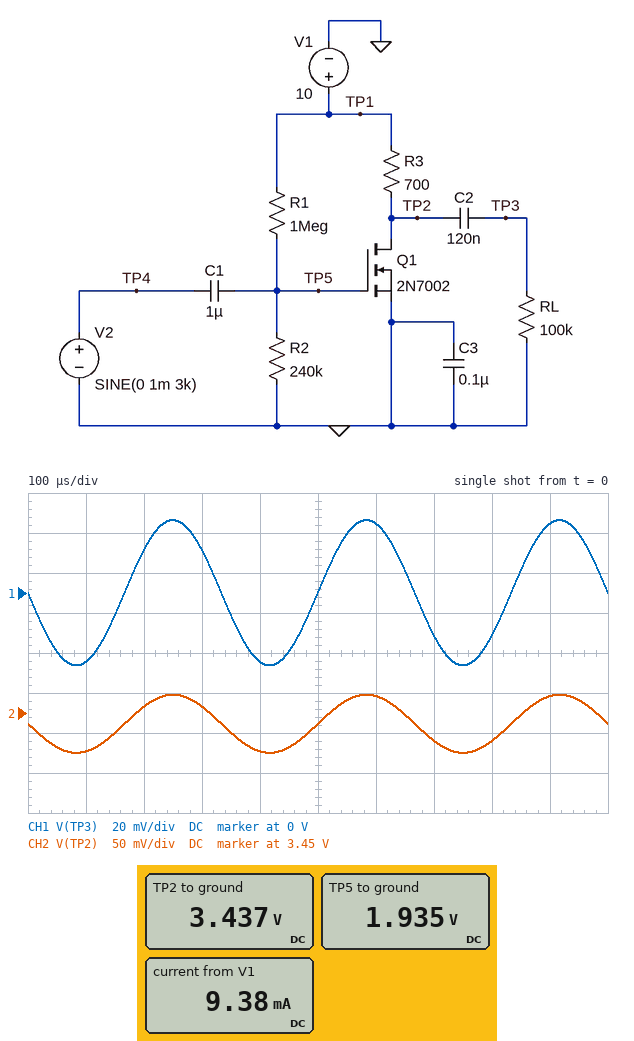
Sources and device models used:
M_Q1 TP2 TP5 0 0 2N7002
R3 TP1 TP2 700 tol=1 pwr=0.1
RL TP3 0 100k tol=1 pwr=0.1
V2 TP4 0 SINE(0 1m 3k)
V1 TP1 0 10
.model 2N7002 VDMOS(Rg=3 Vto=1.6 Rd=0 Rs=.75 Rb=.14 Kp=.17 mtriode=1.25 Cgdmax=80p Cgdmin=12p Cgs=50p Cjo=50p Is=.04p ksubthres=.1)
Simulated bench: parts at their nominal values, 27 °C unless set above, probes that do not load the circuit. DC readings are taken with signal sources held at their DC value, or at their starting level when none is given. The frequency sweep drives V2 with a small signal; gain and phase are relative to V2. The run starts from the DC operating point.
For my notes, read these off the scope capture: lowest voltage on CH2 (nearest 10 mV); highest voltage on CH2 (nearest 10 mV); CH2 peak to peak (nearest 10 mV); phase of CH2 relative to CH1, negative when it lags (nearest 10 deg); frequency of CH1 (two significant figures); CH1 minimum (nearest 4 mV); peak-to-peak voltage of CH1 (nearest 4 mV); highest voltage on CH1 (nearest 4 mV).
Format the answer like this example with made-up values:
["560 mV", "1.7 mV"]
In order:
["3.40 V", "3.47 V", "70 mV", "0 deg", "3.0 kHz", "-36 mV", "72 mV", "36 mV"]
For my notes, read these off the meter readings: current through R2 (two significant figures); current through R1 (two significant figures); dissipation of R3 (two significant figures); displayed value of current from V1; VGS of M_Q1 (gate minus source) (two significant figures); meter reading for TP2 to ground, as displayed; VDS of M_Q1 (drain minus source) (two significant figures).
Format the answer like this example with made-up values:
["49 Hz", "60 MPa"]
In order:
["8.1 µA", "8.1 µA", "62 mW", "9.38 mA", "1.9 V", "3.437 V", "3.4 V"]
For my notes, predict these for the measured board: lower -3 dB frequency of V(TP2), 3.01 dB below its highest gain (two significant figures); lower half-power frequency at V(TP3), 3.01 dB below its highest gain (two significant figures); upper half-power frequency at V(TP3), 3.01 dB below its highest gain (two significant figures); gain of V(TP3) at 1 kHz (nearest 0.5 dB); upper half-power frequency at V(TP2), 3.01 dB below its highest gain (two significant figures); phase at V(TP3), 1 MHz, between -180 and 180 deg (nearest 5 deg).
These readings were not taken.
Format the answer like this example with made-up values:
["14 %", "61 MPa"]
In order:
["810 mHz", "13 Hz", "4.3 MHz", "31.0 dB", "4.3 MHz", "165 deg"]
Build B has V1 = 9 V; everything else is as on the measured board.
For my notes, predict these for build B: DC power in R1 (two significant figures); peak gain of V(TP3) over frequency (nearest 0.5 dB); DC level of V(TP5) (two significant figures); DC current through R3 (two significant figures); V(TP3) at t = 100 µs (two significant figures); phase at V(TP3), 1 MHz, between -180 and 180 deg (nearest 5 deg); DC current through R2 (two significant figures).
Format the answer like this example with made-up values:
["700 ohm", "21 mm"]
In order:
["53 µW", "23.5 dB", "1.7 V", "2.2 mA", "-14 mV", "170 deg", "7.3 µA"]
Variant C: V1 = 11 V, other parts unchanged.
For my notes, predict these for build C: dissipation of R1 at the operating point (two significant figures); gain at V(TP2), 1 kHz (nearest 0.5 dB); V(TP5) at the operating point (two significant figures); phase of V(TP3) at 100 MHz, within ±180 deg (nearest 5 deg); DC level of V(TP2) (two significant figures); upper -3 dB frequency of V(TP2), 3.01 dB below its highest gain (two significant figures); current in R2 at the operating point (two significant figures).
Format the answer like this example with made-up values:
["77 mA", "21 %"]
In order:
["79 µW", "-4.5 dB", "2.1 V", "60 deg", "190 mV", "710 MHz", "8.9 µA"]
